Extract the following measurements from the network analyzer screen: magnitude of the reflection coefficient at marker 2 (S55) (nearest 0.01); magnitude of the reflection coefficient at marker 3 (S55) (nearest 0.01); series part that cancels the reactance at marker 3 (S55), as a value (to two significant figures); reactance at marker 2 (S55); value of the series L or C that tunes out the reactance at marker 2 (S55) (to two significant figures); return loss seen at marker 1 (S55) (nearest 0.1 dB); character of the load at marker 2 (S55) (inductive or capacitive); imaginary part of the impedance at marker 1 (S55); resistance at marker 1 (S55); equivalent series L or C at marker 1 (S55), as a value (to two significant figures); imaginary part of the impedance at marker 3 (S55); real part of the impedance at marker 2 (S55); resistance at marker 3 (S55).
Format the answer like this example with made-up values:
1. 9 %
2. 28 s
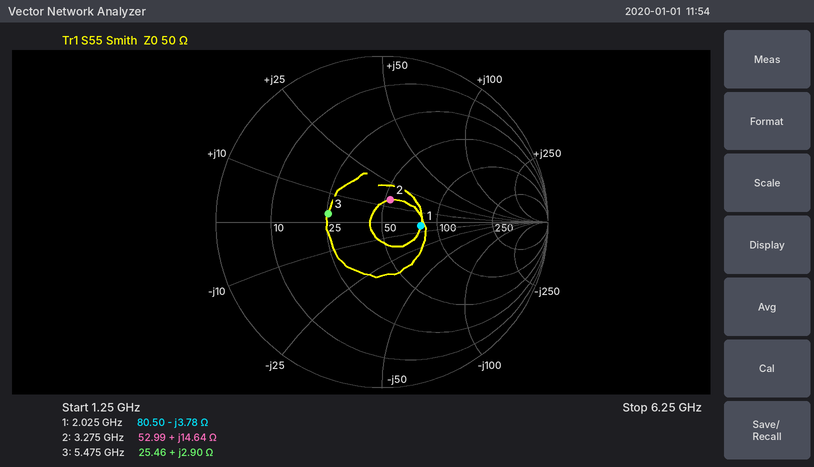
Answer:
1. 0.14
2. 0.33
3. 10 pF
4. +14.64 Ω
5. 3.3 pF
6. 12.6 dB
7. inductive
8. -3.78 Ω
9. 80.50 Ω
10. 21 pF
11. +2.90 Ω
12. 52.99 Ω
13. 25.46 Ω
